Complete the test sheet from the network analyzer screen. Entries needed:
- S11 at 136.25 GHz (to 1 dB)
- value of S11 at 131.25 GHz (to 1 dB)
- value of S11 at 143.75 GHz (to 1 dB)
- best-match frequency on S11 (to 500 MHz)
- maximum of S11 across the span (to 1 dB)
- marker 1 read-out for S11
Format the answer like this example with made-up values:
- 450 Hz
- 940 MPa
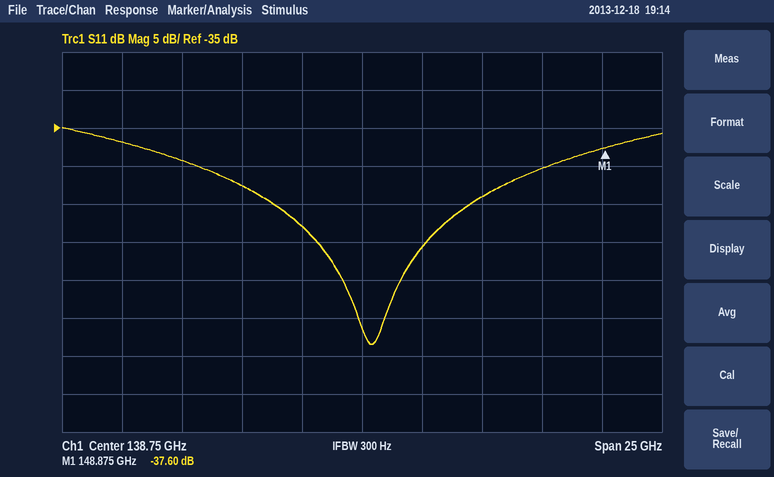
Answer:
- -48 dB
- -39 dB
- -44 dB
- 139.0 GHz
- -35 dB
- -37.60 dB
